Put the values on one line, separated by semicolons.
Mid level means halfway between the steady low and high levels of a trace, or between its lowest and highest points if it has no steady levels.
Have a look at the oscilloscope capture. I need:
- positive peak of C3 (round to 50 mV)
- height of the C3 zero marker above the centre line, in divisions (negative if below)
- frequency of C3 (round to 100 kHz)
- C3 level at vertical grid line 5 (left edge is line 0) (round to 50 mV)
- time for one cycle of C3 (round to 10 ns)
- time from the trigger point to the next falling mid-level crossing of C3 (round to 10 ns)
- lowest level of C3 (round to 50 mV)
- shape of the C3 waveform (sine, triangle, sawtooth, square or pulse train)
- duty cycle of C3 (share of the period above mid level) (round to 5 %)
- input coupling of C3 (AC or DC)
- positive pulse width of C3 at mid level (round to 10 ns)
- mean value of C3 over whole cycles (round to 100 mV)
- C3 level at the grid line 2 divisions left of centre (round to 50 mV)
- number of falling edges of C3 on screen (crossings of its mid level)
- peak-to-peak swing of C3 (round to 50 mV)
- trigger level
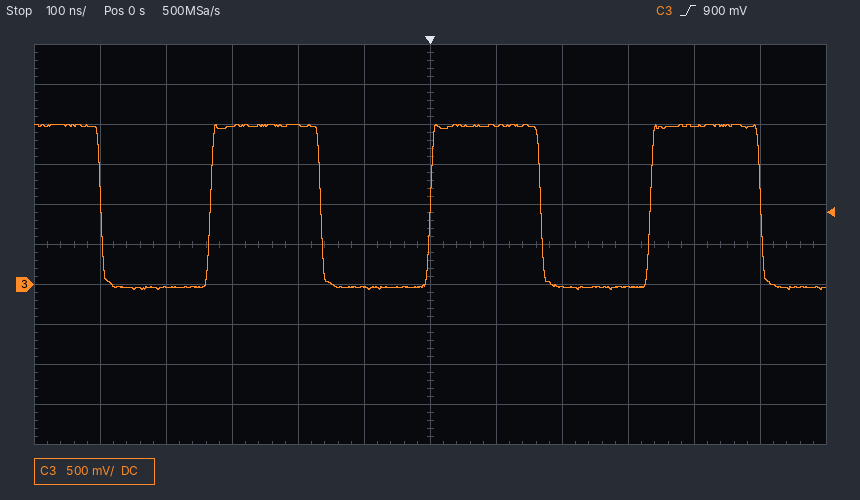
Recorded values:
2.00 V; -1.0 div; 3.0 MHz; -50 mV; 330 ns; 170 ns; -50 mV; square; 50 %; DC; 170 ns; 1.0 V; 2.00 V; 4; 2.05 V; 900 mV
